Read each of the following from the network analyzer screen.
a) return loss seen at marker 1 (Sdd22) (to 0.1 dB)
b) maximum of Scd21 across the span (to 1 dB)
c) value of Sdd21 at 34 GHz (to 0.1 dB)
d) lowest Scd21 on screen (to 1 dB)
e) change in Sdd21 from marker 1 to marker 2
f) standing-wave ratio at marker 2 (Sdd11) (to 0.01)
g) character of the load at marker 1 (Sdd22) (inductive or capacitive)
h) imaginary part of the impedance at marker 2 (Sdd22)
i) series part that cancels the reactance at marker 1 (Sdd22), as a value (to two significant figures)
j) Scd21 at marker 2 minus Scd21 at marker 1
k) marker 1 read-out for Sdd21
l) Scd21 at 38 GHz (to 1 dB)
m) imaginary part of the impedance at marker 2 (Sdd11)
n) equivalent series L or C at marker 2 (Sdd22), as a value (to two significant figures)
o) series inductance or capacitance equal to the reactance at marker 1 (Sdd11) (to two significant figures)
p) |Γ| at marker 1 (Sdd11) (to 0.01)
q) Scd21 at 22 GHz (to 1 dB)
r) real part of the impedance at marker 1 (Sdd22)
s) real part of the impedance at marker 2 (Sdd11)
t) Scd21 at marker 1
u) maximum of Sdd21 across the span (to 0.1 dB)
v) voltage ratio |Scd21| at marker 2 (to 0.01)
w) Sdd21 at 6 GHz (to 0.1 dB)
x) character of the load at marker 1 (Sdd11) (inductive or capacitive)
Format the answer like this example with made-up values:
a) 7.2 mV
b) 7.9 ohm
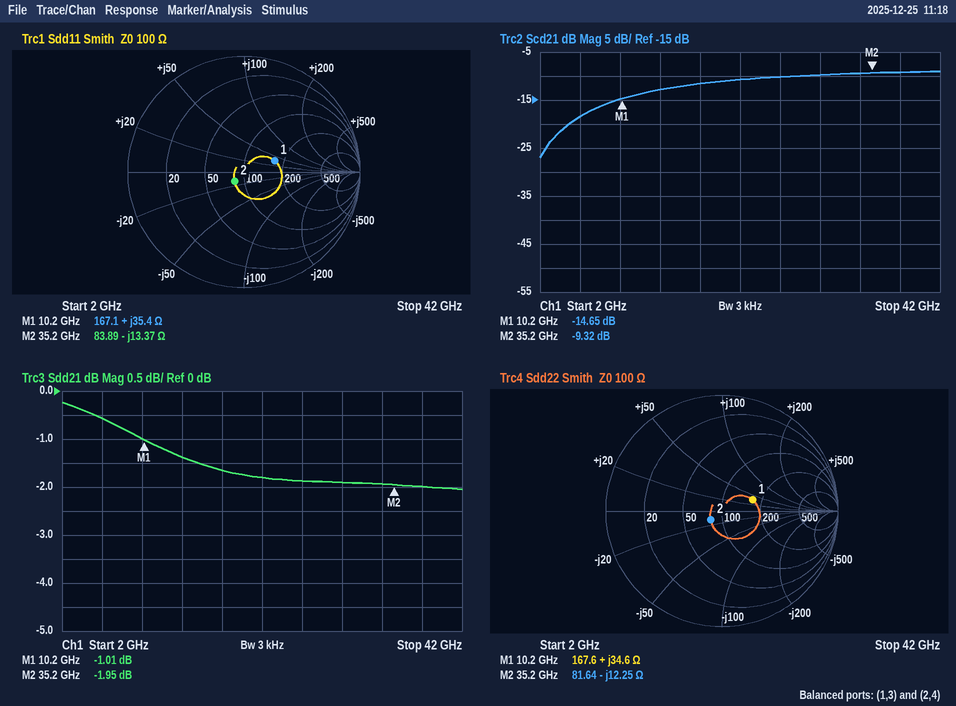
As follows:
a) 11.0 dB
b) -9 dB
c) -1.9 dB
d) -27 dB
e) -0.94 dB
f) 1.26
g) inductive
h) -12.25 Ω
i) 450 fF
j) 5.33 dB
k) -1.01 dB
l) -9 dB
m) -13.37 Ω
n) 370 fF
o) 550 pH
p) 0.28
q) -11 dB
r) 167.6 Ω
s) 83.89 Ω
t) -14.65 dB
u) -0.2 dB
v) 0.34
w) -0.6 dB
x) inductive
